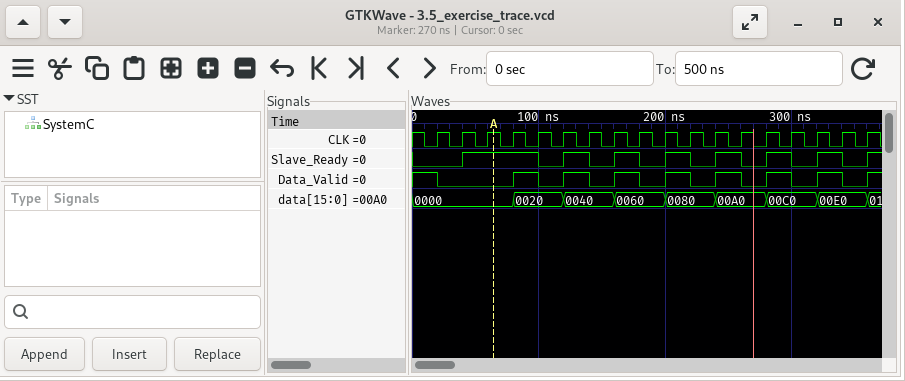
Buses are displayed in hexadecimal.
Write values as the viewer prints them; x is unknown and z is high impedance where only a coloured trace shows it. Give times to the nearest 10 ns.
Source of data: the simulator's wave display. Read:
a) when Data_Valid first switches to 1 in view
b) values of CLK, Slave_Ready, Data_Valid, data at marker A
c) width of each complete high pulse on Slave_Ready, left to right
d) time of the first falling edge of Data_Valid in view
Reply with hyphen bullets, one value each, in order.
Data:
- 80 ns
- CLK=1, Slave_Ready=1, Data_Valid=0, data=0000
- 60 ns, 20 ns, 20 ns, 20 ns, 20 ns, 20 ns, 20 ns
- 20 ns
